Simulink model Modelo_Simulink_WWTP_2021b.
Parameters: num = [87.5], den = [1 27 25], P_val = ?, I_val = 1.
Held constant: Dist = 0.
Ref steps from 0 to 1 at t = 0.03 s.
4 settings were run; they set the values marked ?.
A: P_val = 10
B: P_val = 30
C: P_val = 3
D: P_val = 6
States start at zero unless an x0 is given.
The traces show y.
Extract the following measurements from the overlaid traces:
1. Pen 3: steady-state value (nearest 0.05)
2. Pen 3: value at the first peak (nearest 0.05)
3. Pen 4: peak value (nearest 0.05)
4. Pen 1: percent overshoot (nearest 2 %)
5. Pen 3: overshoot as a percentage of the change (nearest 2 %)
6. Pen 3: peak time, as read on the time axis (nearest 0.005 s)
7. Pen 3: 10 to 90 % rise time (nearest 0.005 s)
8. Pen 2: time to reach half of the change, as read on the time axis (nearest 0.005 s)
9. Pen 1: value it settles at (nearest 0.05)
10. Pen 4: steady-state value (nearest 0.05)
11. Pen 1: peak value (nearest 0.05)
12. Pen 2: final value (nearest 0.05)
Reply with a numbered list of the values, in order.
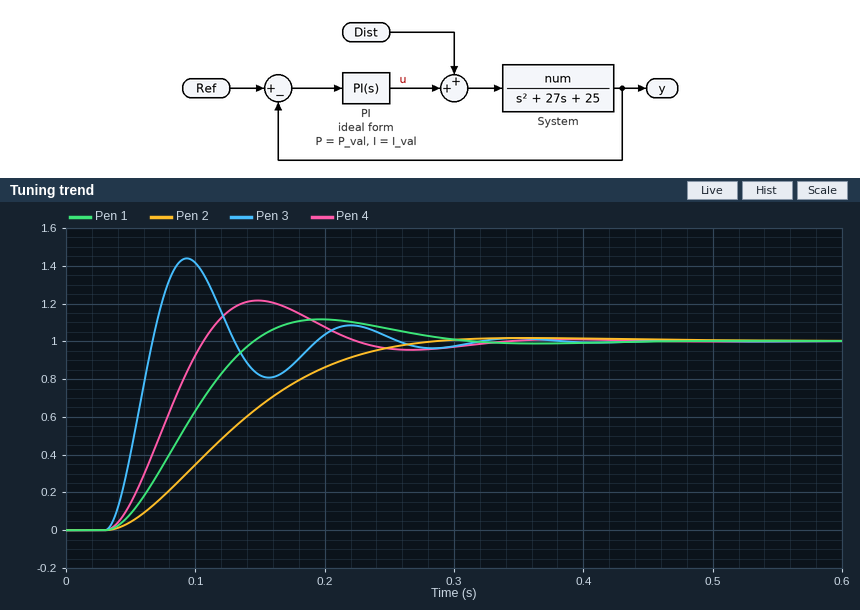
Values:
1. 1.00
2. 1.45
3. 1.20
4. 12 %
5. 44 %
6. 0.095 s
7. 0.025 s
8. 0.125 s
9. 1.00
10. 1.00
11. 1.10
12. 1.00
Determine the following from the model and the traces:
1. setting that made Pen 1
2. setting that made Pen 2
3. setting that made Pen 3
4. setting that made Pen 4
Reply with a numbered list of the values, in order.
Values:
1. D
2. C
3. B
4. A
